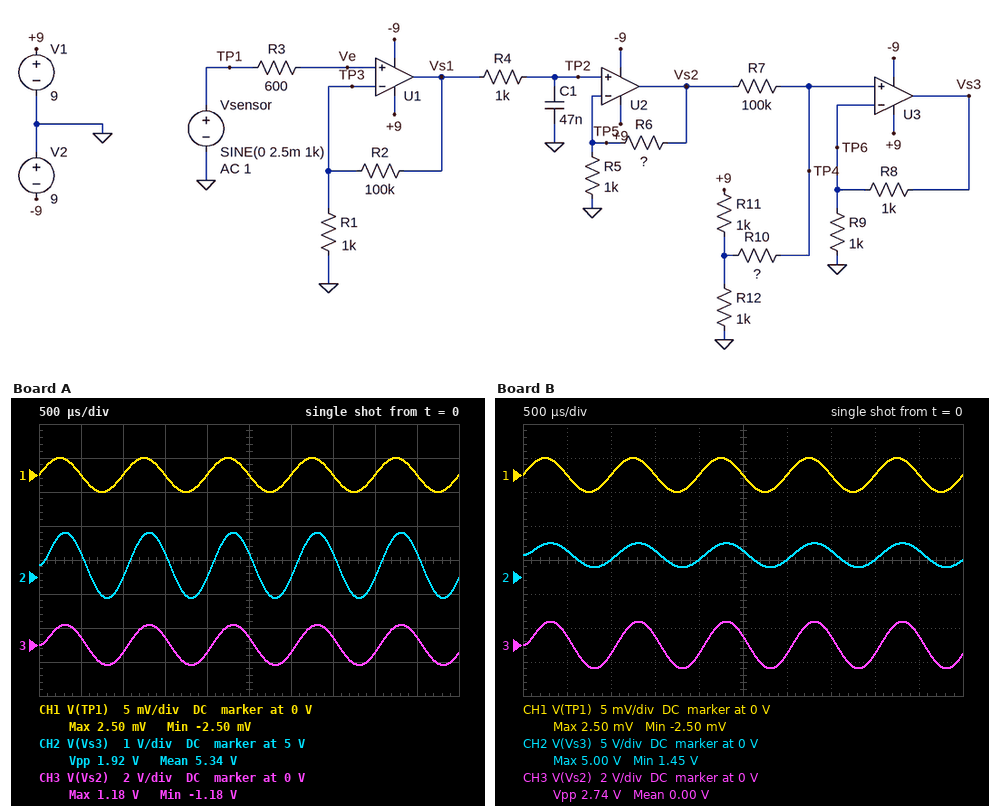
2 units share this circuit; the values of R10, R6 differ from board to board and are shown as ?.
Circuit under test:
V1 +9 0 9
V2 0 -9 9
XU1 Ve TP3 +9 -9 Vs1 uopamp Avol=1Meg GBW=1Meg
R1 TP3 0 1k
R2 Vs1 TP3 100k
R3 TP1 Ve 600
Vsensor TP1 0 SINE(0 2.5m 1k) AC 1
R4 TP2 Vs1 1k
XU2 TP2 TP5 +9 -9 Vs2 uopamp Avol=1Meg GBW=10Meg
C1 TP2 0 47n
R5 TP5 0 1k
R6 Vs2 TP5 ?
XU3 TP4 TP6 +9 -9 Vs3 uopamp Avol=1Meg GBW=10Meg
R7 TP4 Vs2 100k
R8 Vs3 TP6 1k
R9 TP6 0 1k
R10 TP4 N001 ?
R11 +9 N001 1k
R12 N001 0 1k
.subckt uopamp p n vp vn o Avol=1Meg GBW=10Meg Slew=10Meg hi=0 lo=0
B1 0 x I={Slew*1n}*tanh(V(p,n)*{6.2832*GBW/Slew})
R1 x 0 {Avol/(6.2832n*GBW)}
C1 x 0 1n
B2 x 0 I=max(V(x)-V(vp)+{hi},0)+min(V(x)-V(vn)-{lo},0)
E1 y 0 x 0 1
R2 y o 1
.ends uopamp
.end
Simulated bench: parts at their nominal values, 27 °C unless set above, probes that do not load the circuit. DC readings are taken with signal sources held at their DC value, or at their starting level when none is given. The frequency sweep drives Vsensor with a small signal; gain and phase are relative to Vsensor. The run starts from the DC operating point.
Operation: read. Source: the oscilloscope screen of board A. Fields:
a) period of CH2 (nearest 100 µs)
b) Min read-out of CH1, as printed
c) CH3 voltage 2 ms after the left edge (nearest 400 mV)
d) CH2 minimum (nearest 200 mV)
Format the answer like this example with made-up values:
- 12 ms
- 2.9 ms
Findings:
- 1.0 ms
- -2.50 mV
- -400 mV
- 4.4 V
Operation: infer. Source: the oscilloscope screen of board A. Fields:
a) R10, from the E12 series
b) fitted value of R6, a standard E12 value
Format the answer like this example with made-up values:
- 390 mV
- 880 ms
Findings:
- 68 kΩ
- 3.9 kΩ
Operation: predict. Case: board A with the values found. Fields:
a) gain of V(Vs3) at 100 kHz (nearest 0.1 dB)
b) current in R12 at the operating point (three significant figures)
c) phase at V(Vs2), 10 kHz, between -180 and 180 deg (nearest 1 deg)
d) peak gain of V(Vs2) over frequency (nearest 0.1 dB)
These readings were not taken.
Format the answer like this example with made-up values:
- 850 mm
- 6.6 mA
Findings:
- 2.5 dB
- 4.49 mA
- -117 deg
- 53.9 dB
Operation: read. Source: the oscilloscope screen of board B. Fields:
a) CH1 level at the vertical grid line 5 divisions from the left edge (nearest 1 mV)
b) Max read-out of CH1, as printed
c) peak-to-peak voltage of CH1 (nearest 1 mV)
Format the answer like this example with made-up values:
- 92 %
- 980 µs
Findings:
- 0 V
- 2.50 mV
- 5 mV
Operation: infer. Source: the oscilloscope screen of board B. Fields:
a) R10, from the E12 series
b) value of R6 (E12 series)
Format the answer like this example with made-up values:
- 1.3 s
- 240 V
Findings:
- 180 kΩ
- 4.7 kΩ
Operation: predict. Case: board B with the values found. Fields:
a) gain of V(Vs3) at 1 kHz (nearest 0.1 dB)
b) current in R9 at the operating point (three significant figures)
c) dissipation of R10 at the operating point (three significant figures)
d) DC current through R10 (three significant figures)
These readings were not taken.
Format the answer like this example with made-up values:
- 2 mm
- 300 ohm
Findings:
- 57.0 dB
- 1.60 mA
- 46.3 µW
- 16.0 µA
